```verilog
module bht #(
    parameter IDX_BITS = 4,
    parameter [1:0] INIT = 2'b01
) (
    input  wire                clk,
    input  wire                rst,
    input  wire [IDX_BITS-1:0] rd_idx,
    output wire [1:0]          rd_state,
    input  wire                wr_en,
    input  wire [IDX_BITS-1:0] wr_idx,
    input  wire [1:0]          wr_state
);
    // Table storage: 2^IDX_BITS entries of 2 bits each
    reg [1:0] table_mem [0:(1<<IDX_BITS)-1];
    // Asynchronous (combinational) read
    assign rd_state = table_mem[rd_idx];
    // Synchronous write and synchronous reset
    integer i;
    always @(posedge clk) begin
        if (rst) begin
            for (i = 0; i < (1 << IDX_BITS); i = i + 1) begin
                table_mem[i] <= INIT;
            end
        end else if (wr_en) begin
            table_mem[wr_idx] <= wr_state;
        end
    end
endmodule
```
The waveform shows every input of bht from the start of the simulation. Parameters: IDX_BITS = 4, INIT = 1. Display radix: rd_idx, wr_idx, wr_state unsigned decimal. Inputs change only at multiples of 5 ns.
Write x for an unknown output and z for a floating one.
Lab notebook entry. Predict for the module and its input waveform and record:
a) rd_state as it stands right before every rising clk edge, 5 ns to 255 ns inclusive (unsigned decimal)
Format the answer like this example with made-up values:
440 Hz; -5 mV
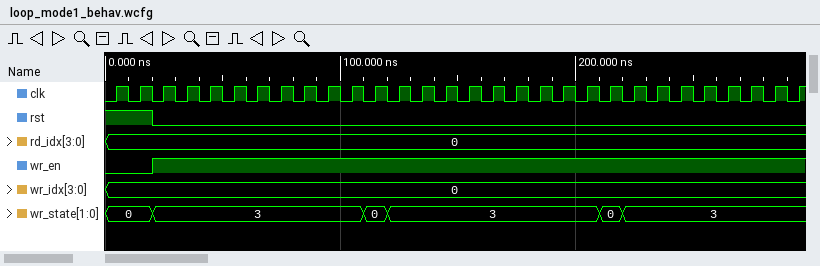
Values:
x, 1, 1, 3, 3, 3, 3, 3, 3, 3, 3, 3, 0, 3, 3, 3, 3, 3, 3, 3, 3, 3, 0, 3, 3, 3
